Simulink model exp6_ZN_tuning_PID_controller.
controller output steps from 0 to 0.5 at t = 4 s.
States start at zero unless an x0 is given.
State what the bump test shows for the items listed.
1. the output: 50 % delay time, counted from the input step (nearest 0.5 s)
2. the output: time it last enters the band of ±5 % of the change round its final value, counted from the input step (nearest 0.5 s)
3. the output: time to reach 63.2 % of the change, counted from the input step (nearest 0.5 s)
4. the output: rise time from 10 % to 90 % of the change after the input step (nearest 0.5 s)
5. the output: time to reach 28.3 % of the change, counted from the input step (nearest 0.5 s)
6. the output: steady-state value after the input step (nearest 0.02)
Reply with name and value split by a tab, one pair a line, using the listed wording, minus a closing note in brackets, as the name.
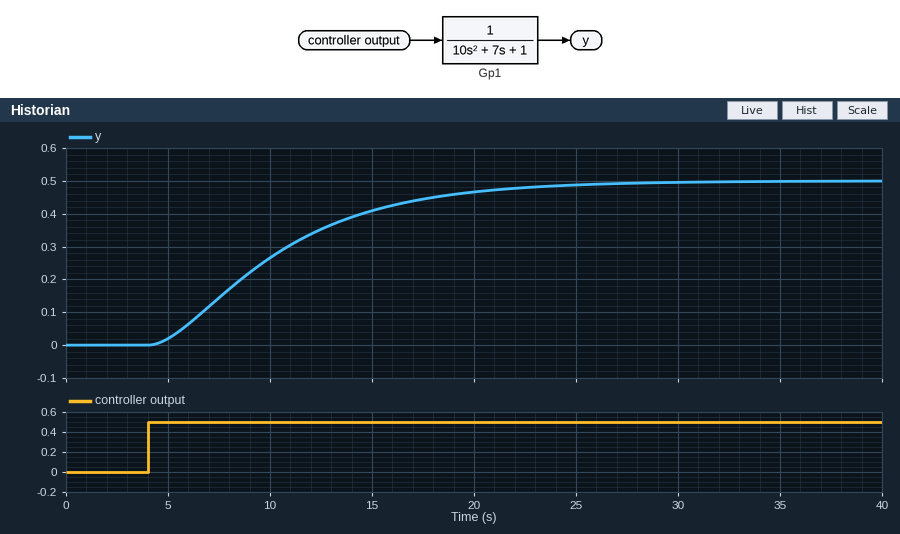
the output: 50 % delay time, counted from the input step	5.5 s
the output: time it last enters the band of ±5 % of the change round its final value, counted from the input step	17.5 s
the output: time to reach 63.2 % of the change, counted from the input step	7.5 s
the output: rise time from 10 % to 90 % of the change after the input step	12.5 s
the output: time to reach 28.3 % of the change, counted from the input step	3.5 s
the output: steady-state value after the input step	0.50
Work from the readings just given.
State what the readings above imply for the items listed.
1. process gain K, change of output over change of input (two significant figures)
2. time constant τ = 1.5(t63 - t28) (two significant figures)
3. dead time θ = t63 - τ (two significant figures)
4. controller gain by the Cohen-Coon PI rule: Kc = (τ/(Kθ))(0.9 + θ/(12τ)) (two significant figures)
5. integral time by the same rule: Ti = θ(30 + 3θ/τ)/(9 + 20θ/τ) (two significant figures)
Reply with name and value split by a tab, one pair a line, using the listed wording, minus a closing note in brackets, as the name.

process gain K, change of output over change of input	1.0
time constant τ = 1.5(t63 - t28)	6.0 s
dead time θ = t63 - τ	1.5 s
controller gain by the Cohen-Coon PI rule: Kc = (τ/(Kθ))(0.9 + θ/(12τ))	3.7
integral time by the same rule: Ti = θ(30 + 3θ/τ)/(9 + 20θ/τ)	3.3 s
